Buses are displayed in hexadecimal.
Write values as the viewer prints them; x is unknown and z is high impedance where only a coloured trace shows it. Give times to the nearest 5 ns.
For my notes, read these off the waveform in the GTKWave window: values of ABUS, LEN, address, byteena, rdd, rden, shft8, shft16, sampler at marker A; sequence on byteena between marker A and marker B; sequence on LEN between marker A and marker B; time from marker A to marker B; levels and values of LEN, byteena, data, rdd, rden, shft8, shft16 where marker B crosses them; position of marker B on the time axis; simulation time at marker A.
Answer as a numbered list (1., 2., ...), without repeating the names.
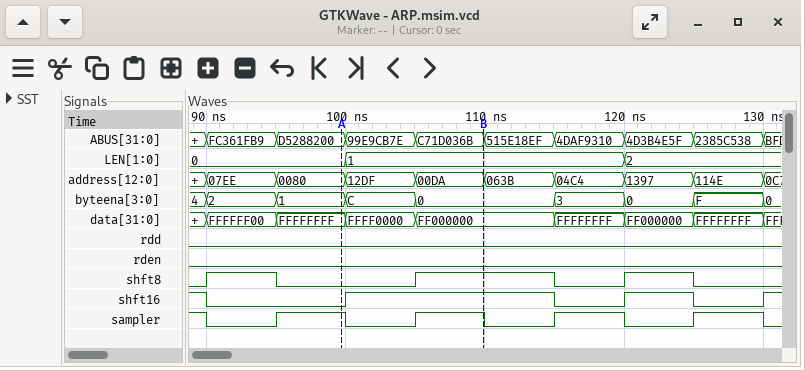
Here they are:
1. ABUS=D5288200, LEN=0, address=0080, byteena=1, rdd=0, rden=0, shft8=0, shft16=0, sampler=1
2. 1, C, 0
3. 0, 1
4. 10 ns
5. LEN=1, byteena=0, data=FF000000, rdd=0, rden=0, shft8=1, shft16=1
6. 110 ns
7. 100 ns
